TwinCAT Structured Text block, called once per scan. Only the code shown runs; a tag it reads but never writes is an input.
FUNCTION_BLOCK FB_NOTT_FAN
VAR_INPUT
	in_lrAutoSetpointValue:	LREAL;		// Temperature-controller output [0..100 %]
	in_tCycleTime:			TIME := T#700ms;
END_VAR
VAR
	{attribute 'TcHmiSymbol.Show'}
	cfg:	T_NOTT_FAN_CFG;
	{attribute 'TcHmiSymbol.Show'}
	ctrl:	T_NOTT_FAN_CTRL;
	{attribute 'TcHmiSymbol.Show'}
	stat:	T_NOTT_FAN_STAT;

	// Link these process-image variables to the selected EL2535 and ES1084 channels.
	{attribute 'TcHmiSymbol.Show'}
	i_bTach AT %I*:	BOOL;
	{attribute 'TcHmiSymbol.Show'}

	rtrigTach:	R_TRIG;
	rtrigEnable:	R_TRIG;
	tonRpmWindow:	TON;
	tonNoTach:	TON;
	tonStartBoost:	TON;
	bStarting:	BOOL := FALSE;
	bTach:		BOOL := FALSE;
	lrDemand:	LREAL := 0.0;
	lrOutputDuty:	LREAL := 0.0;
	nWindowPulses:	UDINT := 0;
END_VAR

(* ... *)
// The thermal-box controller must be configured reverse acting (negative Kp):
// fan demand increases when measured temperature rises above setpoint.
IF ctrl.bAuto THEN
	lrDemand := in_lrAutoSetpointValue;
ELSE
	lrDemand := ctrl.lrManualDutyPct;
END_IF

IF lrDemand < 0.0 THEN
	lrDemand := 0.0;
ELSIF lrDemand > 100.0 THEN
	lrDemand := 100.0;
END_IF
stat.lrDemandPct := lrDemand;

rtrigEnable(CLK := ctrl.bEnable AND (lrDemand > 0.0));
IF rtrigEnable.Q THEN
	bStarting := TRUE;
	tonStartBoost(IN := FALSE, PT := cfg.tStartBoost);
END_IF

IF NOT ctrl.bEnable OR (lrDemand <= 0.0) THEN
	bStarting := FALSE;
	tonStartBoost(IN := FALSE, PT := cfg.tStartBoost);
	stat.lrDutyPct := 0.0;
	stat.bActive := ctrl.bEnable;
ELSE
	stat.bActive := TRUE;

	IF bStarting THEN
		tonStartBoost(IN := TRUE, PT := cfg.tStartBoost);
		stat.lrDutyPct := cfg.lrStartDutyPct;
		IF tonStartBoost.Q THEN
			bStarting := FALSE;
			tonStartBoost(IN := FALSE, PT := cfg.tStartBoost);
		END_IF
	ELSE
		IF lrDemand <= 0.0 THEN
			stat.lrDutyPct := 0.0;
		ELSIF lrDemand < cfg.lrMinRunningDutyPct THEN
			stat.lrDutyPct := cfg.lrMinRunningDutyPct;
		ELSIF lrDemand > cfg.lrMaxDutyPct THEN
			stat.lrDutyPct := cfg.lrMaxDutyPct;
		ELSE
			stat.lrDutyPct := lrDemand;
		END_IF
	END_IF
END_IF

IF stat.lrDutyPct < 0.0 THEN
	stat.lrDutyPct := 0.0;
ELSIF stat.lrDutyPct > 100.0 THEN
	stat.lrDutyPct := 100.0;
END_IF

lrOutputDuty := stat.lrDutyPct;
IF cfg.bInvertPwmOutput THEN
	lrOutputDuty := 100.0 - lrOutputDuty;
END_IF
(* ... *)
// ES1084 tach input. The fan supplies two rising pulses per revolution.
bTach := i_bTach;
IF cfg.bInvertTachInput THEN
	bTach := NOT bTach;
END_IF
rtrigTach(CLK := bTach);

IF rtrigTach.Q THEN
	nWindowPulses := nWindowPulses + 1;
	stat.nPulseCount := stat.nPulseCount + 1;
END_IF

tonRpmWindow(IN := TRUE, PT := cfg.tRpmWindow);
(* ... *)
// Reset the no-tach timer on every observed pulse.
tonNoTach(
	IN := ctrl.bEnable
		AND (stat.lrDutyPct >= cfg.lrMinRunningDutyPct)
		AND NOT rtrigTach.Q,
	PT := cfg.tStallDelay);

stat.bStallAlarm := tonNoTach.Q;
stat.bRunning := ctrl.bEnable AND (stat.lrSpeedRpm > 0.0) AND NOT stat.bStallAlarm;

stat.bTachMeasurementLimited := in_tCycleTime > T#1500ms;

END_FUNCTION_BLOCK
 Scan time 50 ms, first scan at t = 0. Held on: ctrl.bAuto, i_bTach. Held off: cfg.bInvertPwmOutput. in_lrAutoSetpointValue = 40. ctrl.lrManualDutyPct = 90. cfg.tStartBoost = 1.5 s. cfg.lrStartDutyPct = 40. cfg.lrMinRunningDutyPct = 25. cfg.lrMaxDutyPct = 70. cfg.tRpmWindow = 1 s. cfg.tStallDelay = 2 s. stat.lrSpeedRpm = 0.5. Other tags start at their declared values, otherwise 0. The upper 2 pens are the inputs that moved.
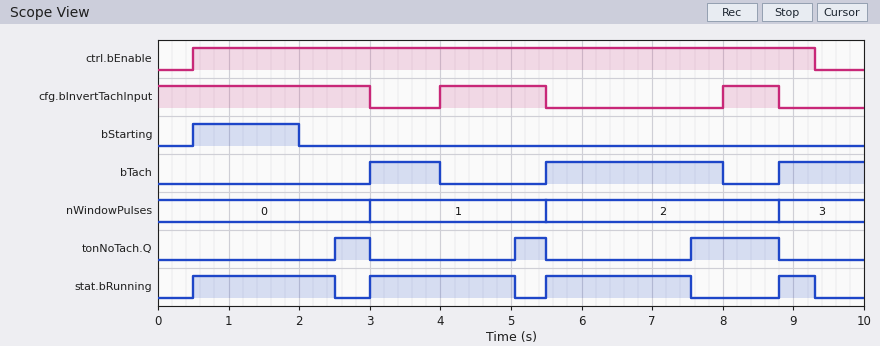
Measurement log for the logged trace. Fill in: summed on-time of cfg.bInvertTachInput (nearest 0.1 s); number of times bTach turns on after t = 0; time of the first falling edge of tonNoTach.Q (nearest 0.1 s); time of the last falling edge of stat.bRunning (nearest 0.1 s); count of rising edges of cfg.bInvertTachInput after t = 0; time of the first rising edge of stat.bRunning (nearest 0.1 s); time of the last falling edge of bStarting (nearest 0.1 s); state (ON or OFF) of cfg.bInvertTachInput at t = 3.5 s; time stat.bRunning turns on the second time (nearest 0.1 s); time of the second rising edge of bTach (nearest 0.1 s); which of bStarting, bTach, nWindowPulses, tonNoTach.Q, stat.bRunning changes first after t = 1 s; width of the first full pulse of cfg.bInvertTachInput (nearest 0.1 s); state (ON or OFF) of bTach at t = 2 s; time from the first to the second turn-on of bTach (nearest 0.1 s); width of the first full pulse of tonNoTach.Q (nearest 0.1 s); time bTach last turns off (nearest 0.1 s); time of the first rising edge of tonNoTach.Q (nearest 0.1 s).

5.3 s
3
3.0 s
9.3 s
2
0.5 s
2.0 s
OFF
3.0 s
5.5 s
bStarting
1.5 s
OFF
2.5 s
0.5 s
8.0 s
2.5 s
